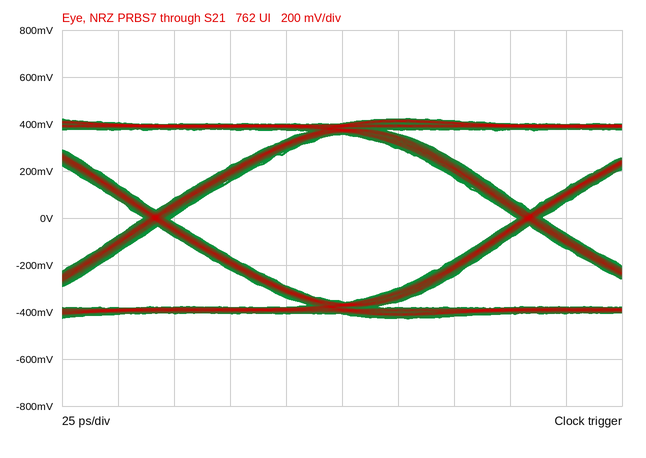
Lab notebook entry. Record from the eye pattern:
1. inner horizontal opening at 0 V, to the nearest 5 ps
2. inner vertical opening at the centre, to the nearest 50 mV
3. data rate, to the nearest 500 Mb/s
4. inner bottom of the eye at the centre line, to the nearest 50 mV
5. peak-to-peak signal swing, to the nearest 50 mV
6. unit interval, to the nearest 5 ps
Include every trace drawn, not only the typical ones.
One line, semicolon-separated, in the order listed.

155 ps; 700 mV; 6.0 Gb/s; -350 mV; 850 mV; 165 ps
